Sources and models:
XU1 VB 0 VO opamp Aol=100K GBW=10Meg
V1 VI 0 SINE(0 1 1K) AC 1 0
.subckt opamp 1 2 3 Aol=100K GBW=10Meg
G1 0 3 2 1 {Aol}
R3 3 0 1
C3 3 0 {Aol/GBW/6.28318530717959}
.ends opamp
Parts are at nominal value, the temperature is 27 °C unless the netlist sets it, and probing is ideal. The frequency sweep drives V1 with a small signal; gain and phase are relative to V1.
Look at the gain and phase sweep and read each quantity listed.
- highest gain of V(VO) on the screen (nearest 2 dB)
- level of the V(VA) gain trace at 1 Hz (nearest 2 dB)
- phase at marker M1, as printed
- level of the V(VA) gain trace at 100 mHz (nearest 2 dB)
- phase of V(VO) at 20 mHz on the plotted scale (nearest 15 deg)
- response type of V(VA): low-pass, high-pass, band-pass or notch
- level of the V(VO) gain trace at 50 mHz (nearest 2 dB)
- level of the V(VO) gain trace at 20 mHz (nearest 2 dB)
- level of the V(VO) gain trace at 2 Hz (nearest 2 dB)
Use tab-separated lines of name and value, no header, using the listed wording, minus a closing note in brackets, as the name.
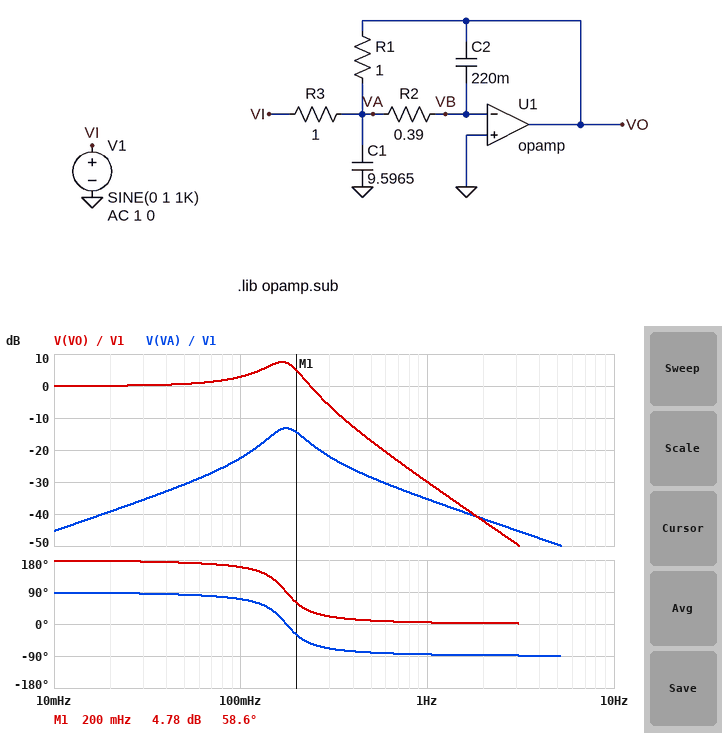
highest gain of V(VO) on the screen	8 dB
level of the V(VA) gain trace at 1 Hz	-36 dB
phase at marker M1, as printed	58.6 deg
level of the V(VA) gain trace at 100 mHz	-22 dB
phase of V(VO) at 20 mHz on the plotted scale	180 deg
response type of V(VA): low-pass, high-pass, band-pass or notch	band-pass
level of the V(VO) gain trace at 50 mHz	0 dB
level of the V(VO) gain trace at 20 mHz	0 dB
level of the V(VO) gain trace at 2 Hz	-42 dB
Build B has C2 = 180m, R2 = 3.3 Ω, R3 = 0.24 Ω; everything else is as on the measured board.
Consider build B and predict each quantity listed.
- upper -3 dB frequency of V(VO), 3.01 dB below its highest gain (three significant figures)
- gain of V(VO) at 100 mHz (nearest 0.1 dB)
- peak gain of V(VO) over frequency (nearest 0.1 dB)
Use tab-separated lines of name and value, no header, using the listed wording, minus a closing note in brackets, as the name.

upper -3 dB frequency of V(VO), 3.01 dB below its highest gain	69.0 mHz
gain of V(VO) at 100 mHz	4.8 dB
peak gain of V(VO) over frequency	12.4 dB
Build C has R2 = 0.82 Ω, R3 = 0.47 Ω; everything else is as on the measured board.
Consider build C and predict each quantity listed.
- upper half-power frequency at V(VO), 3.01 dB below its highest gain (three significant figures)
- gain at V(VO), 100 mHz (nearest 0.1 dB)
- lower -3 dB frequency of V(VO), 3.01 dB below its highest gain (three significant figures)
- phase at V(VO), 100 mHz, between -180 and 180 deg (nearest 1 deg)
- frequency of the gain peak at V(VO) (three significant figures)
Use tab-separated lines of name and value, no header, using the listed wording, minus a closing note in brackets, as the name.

upper half-power frequency at V(VO), 3.01 dB below its highest gain	143 mHz
gain at V(VO), 100 mHz	11.2 dB
lower -3 dB frequency of V(VO), 3.01 dB below its highest gain	60.9 mHz
phase at V(VO), 100 mHz, between -180 and 180 deg	123 deg
frequency of the gain peak at V(VO)	110 mHz
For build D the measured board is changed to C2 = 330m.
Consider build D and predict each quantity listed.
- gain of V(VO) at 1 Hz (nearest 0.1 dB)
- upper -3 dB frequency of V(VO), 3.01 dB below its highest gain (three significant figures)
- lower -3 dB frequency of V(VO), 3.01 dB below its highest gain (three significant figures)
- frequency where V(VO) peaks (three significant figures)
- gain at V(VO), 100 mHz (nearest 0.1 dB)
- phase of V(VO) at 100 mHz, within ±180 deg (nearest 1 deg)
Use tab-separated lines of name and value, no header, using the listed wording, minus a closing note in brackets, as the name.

gain of V(VO) at 1 Hz	-33.6 dB
upper -3 dB frequency of V(VO), 3.01 dB below its highest gain	168 mHz
lower -3 dB frequency of V(VO), 3.01 dB below its highest gain	84.8 mHz
frequency where V(VO) peaks	133 mHz
gain at V(VO), 100 mHz	4.0 dB
phase of V(VO) at 100 mHz, within ±180 deg	144 deg
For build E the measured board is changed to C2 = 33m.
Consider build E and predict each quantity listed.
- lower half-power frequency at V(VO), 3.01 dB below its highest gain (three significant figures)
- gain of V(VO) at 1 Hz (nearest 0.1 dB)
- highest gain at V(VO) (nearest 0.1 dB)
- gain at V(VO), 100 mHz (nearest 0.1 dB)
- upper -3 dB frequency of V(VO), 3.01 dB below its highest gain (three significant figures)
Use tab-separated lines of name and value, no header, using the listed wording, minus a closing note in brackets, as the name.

lower half-power frequency at V(VO), 3.01 dB below its highest gain	410 mHz
gain of V(VO) at 1 Hz	-11.8 dB
highest gain at V(VO)	15.5 dB
gain at V(VO), 100 mHz	0.4 dB
upper -3 dB frequency of V(VO), 3.01 dB below its highest gain	486 mHz
